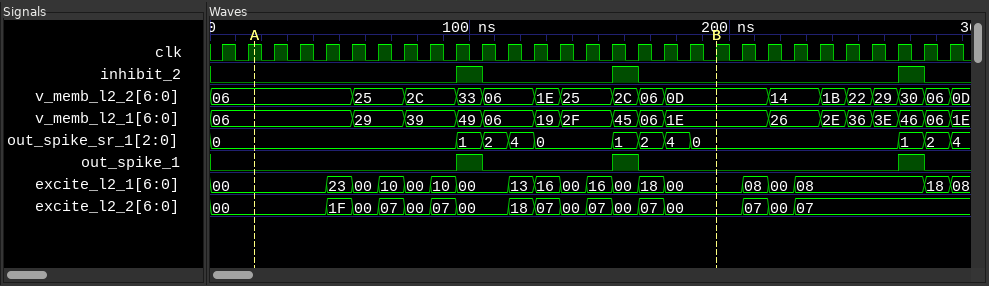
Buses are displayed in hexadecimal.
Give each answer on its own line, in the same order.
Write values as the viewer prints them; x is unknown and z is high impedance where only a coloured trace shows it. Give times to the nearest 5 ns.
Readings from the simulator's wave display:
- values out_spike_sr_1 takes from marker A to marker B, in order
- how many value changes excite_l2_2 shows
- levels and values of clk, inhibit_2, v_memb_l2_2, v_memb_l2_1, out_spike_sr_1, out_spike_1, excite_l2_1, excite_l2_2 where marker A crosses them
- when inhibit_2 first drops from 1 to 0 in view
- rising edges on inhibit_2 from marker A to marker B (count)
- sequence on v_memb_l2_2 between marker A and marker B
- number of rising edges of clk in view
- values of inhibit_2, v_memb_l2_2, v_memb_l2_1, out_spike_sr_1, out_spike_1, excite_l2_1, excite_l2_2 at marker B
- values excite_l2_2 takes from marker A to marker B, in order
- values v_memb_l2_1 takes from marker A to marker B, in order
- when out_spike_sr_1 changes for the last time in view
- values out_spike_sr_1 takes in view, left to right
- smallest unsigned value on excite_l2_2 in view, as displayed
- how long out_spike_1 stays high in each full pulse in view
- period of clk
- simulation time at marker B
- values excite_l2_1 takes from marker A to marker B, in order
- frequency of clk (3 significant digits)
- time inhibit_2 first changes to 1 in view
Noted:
0, 1, 2, 4, 0, 1, 2, 4, 0
16
clk=1, inhibit_2=0, v_memb_l2_2=06, v_memb_l2_1=06, out_spike_sr_1=0, out_spike_1=0, excite_l2_1=00, excite_l2_2=00
105 ns
2
06, 25, 2C, 33, 06, 1E, 25, 2C, 06, 0D
29
inhibit_2=0, v_memb_l2_2=0D, v_memb_l2_1=1E, out_spike_sr_1=0, out_spike_1=0, excite_l2_1=00, excite_l2_2=00
00, 1F, 00, 07, 00, 07, 00, 18, 07, 00, 07, 00, 07, 00
06, 29, 39, 49, 06, 19, 2F, 45, 06, 1E
285 ns
0, 1, 2, 4, 0, 1, 2, 4, 0, 1, 2, 4
00
10 ns, 10 ns, 10 ns
10 ns
195 ns
00, 23, 00, 10, 00, 10, 00, 13, 16, 00, 16, 00, 18, 00
100 MHz
95 ns
